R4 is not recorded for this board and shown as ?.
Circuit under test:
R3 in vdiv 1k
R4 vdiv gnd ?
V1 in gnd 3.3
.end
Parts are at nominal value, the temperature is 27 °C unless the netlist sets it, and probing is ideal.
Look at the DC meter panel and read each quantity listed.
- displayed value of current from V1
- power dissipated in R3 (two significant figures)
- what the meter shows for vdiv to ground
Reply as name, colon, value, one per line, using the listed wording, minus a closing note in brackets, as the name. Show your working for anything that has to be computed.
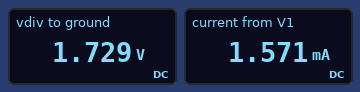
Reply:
displayed value of current from V1: 1.571 mA
power dissipated in R3: (3.3 V - 1.729 V)^2 / 1 kΩ = 2.5 mW
what the meter shows for vdiv to ground: 1.729 V
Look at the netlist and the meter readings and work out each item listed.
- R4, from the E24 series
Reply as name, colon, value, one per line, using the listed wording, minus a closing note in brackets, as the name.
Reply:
R4, from the E24 series: 1.1 kΩ
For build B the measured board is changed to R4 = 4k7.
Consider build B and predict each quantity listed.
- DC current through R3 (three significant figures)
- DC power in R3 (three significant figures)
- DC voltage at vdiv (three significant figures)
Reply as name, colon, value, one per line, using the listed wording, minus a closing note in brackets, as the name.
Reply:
DC current through R3: 579 µA
DC power in R3: 335 µW
DC voltage at vdiv: 2.72 V
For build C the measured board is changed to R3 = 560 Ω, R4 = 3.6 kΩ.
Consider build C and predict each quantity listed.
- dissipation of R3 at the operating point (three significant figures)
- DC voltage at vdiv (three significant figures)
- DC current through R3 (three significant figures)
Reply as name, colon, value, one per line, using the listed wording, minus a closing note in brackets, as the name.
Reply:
dissipation of R3 at the operating point: 352 µW
DC voltage at vdiv: 2.86 V
DC current through R3: 793 µA
